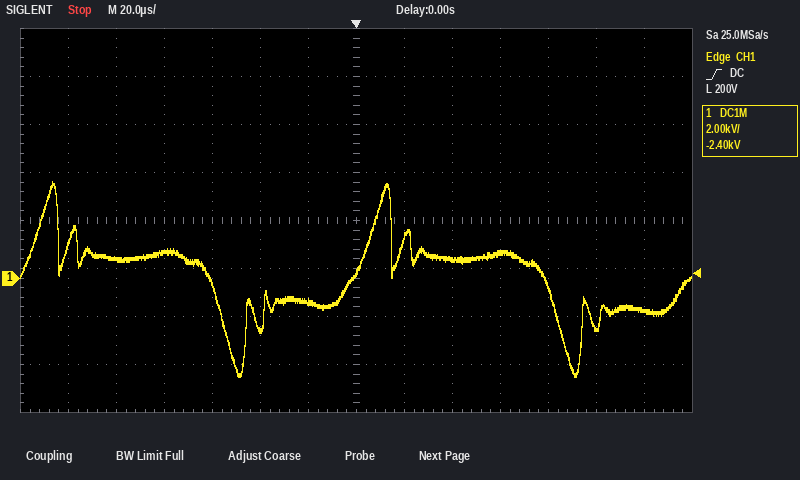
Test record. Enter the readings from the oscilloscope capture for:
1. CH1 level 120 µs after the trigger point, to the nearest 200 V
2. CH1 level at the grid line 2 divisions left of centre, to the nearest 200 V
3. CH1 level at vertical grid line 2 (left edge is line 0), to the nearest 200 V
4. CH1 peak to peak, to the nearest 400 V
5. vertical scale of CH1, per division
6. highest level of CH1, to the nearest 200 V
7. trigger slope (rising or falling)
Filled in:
-1.4 kV
-2.2 kV
800 V
8.0 kV
2 kV
4.0 kV
rising
